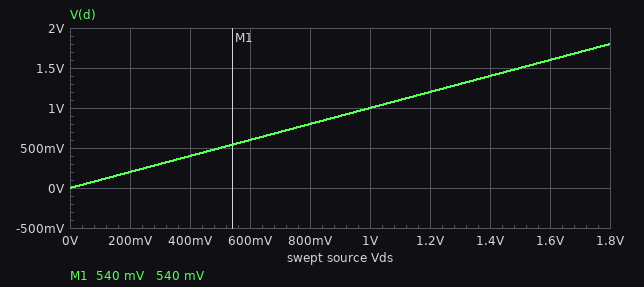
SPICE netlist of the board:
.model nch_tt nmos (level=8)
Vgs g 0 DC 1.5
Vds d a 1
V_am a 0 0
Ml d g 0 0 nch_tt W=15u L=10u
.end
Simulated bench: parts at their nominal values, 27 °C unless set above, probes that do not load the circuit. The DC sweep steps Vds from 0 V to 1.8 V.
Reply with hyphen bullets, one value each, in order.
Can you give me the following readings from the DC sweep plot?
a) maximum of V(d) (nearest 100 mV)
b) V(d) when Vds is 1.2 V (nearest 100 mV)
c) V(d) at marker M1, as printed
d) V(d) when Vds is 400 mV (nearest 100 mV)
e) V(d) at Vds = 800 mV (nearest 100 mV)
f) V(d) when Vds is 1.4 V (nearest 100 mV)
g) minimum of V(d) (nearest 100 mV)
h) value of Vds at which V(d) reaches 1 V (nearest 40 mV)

- 1.8 V
- 1.2 V
- 540 mV
- 400 mV
- 800 mV
- 1.4 V
- 0 V
- 1.00 V
